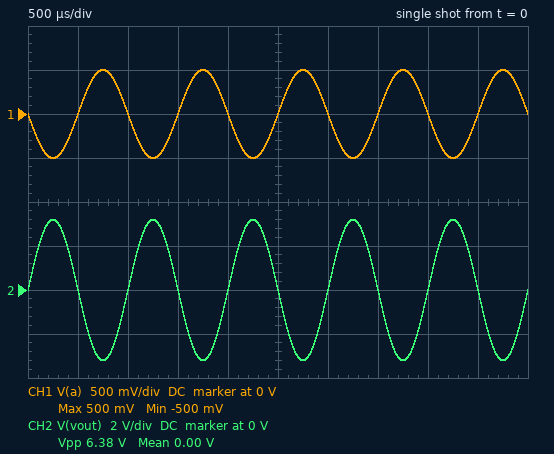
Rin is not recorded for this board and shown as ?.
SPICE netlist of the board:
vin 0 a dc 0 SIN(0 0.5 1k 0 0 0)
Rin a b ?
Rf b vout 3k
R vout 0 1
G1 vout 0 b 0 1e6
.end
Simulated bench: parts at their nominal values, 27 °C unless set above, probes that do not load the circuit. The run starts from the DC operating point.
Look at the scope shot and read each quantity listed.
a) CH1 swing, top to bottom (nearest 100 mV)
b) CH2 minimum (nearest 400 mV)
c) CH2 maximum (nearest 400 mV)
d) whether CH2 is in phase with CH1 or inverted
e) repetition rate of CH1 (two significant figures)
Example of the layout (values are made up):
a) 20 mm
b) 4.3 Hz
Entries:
a) 1.0 V
b) -3.2 V
c) 3.2 V
d) inverted
e) 1.0 kHz
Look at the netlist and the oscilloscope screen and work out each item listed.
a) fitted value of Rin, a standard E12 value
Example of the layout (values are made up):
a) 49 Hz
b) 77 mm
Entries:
a) 470 Ω
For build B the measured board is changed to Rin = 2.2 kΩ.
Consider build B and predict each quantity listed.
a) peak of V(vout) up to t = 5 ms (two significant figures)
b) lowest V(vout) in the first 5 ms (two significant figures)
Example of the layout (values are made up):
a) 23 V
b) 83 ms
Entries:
a) 680 mV
b) -680 mV
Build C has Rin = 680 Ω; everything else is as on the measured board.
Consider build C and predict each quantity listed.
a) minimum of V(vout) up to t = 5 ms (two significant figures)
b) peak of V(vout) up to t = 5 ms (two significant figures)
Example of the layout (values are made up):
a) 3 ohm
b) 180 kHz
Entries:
a) -2.2 V
b) 2.2 V
